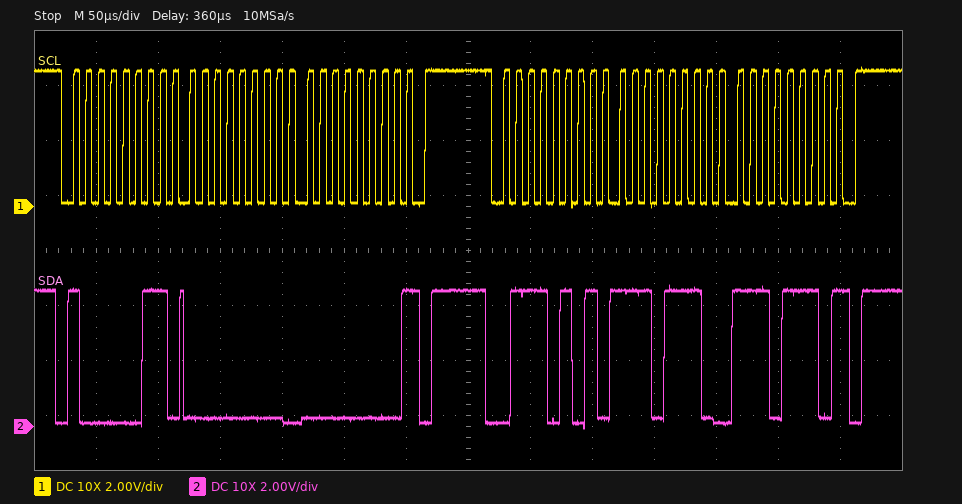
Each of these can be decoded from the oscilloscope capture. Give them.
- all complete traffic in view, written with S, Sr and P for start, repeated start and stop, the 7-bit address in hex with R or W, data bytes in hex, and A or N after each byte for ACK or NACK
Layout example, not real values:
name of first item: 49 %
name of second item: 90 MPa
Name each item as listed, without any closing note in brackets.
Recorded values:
all complete traffic in view, written with S, Sr and P for start, repeated start and stop, the 7-bit address in hex with R or W, data bytes in hex, and A or N after each byte for ACK or NACK: S 41R A 00 A 00 N P S 3AR A EE A EE N P
